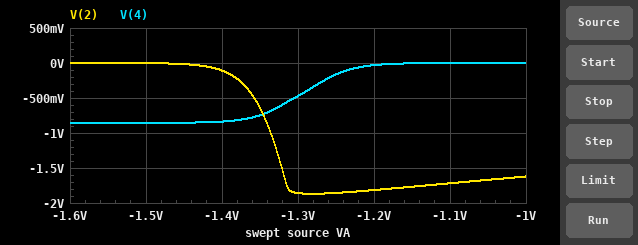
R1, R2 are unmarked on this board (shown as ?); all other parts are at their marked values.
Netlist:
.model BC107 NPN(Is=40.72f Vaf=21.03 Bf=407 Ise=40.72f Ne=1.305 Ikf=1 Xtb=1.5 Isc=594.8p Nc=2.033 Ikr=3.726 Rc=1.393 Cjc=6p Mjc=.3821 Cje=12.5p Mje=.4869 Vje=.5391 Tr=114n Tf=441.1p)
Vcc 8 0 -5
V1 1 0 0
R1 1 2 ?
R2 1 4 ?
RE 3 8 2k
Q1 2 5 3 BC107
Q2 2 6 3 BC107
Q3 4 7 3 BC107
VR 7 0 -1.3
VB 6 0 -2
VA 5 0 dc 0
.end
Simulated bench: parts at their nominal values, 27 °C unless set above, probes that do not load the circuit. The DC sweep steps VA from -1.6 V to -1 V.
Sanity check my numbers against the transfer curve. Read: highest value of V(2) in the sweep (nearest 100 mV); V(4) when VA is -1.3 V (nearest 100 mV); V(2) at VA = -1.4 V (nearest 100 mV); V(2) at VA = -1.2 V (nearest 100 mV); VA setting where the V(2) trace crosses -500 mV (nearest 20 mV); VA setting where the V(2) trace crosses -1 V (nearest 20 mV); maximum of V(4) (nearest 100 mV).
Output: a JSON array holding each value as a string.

["0 V", "-500 mV", "-100 mV", "-1.8 V", "-1.36 V", "-1.34 V", "0 V"]
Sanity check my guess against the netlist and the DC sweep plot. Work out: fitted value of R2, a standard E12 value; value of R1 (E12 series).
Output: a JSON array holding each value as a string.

["560 Ω", "3.3 kΩ"]
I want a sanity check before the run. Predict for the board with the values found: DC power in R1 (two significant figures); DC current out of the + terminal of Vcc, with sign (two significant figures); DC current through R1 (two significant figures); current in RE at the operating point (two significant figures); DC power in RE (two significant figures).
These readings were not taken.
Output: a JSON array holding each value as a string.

["120 µW", "-2.2 mA", "190 µA", "2.2 mA", "9.4 mW"]
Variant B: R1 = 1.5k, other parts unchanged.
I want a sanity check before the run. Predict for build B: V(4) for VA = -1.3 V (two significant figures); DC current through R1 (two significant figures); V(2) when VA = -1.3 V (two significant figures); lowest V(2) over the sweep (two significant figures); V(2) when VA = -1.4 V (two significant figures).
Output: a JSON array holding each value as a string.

["-440 mV", "420 µA", "-1.1 V", "-1.8 V", "-49 mV"]
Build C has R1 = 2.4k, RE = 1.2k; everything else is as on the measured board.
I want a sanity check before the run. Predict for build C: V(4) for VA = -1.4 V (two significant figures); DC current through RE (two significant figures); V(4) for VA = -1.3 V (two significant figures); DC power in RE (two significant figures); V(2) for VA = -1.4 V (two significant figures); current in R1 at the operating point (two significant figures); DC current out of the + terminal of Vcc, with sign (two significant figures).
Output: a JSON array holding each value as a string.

["-1.4 V", "3.6 mA", "-810 mV", "16 mW", "-130 mV", "270 µA", "-3.6 mA"]
